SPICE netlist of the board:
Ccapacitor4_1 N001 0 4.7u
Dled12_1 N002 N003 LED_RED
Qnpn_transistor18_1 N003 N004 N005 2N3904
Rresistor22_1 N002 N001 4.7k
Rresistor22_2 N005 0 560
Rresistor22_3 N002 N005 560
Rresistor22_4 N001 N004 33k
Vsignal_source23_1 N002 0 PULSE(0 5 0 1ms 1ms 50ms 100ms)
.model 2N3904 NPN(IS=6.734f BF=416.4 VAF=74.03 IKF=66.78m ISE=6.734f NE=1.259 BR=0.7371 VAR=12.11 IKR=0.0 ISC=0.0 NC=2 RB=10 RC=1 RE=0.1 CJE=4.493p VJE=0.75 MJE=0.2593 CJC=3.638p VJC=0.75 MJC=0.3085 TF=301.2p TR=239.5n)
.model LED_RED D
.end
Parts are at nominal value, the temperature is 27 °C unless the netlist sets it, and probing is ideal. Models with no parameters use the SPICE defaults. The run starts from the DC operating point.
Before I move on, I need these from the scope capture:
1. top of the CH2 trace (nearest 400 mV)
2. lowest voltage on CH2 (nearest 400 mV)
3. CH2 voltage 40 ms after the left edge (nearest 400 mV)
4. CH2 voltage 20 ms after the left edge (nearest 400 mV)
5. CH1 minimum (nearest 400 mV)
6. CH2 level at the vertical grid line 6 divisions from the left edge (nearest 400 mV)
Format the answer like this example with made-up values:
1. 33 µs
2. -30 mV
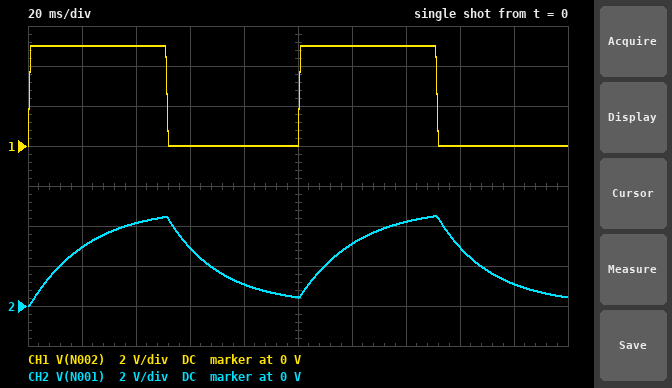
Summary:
1. 4.4 V
2. 0 V
3. 4.0 V
4. 2.8 V
5. 0 V
6. 3.2 V
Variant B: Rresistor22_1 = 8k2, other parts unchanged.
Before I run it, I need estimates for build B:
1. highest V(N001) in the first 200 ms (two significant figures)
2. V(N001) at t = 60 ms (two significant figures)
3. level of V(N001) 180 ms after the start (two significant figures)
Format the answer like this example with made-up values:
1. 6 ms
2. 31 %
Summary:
1. 3.9 V
2. 2.8 V
3. 1.6 V
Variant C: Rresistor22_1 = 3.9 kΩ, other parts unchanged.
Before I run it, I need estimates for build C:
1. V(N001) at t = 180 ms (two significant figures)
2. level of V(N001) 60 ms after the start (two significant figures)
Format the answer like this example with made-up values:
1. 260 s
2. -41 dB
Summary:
1. 870 mV
2. 2.8 V
